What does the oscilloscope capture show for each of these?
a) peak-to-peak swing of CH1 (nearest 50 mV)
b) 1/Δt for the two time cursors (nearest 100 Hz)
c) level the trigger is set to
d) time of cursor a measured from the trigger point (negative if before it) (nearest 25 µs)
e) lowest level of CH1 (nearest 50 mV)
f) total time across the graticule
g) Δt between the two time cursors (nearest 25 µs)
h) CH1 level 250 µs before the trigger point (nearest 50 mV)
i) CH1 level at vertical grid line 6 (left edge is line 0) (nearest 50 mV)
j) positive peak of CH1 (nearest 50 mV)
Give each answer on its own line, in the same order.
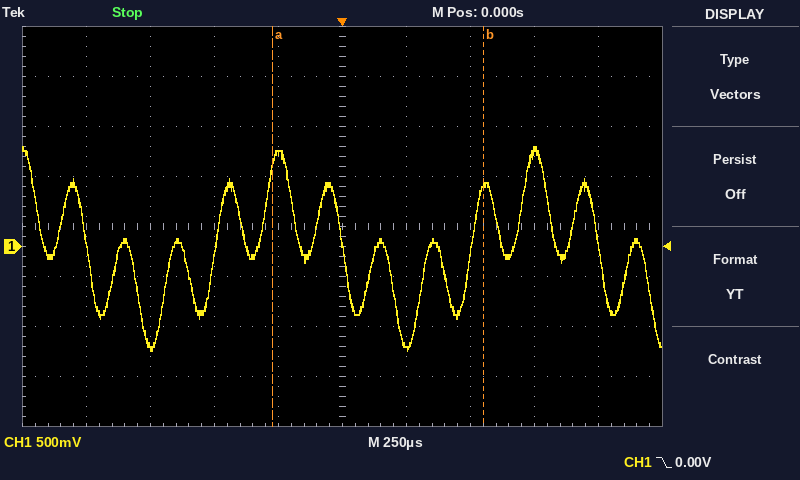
2.05 V
1.2 kHz
0.00 V
-275 µs
-1.05 V
2.5 ms
825 µs
950 mV
-1.00 V
1.00 V
